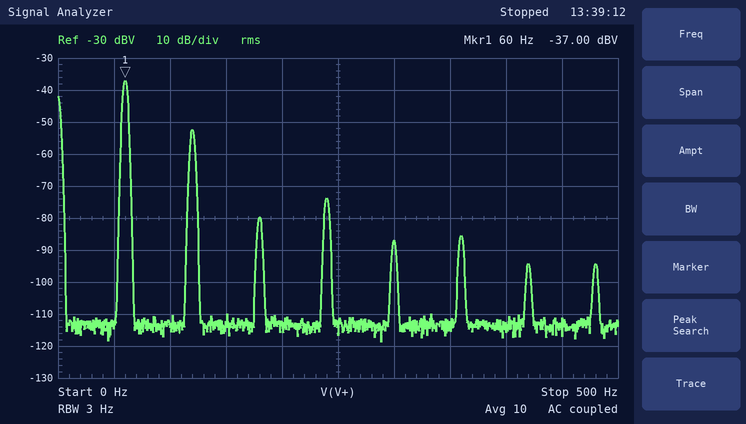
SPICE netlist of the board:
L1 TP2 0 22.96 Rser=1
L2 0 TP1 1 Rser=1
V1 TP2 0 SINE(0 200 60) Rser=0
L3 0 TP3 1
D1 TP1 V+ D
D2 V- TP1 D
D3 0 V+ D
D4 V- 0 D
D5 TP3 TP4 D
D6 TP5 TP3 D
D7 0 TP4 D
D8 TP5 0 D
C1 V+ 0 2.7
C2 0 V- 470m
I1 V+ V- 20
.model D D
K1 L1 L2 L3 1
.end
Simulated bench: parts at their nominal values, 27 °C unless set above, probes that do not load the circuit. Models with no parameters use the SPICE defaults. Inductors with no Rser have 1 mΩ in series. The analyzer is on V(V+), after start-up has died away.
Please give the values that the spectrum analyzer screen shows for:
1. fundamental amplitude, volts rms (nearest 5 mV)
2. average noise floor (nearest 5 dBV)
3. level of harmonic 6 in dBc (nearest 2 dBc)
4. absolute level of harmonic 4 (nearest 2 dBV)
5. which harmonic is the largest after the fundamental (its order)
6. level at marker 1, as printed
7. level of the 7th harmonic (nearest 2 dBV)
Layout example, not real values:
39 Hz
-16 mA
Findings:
15 mV
-115 dBV
-48 dBc
-74 dBV
2
-37.00 dBV
-94 dBV
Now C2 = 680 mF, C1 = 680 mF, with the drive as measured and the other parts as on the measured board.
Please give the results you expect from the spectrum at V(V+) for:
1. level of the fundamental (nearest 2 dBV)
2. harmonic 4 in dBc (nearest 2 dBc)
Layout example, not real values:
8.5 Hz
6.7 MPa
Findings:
-26 dBV
-36 dBc
